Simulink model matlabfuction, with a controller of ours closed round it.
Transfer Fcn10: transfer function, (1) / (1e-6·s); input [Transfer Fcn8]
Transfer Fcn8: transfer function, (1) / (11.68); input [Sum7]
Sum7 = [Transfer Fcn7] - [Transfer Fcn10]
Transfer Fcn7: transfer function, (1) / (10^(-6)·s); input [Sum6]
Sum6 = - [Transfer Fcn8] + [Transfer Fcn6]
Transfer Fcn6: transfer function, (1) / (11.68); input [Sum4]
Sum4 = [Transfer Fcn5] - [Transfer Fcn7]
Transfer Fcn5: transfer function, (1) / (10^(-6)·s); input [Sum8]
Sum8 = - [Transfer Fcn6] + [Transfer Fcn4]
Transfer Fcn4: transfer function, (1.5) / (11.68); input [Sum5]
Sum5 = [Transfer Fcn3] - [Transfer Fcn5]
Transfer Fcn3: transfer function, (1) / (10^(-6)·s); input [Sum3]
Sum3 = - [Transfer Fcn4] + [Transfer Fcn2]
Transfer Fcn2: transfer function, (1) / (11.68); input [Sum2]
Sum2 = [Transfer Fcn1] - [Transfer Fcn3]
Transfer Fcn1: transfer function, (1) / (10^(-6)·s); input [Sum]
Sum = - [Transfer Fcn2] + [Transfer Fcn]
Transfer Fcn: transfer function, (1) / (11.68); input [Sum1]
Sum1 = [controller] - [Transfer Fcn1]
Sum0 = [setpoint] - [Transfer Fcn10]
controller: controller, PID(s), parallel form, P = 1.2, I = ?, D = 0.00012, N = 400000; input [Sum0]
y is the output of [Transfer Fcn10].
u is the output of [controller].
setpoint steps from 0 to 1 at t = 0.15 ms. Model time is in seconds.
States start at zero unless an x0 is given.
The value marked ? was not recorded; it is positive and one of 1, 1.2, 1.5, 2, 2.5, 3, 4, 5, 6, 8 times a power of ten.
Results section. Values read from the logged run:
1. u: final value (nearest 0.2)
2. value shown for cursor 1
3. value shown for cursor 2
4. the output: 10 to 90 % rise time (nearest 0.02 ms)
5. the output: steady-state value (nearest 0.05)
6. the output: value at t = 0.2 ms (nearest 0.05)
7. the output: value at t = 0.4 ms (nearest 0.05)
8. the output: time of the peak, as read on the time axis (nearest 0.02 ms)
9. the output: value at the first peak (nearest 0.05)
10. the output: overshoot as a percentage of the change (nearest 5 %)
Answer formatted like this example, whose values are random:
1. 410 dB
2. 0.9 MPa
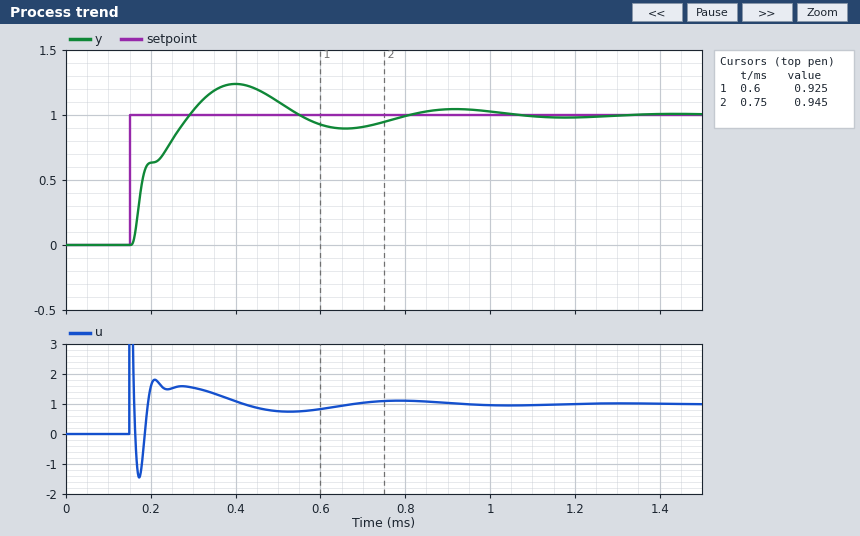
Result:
1. 1.0
2. 0.925
3. 0.945
4. 0.10 ms
5. 1.00
6. 0.65
7. 1.25
8. 0.40 ms
9. 1.25
10. 25 %
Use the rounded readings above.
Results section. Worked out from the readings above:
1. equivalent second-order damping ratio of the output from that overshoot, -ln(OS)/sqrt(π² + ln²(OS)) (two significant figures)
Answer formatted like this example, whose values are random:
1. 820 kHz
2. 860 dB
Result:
1. 0.40
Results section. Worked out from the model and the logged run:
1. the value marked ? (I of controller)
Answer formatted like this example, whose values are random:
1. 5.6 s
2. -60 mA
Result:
1. 40000
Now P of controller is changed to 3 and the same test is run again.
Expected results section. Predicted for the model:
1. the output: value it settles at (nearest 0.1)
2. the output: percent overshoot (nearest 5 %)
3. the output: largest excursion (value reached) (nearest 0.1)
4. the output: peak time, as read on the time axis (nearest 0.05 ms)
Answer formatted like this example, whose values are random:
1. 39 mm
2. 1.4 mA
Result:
1. 1.0
2. 10 %
3. 1.1
4. 0.35 ms
